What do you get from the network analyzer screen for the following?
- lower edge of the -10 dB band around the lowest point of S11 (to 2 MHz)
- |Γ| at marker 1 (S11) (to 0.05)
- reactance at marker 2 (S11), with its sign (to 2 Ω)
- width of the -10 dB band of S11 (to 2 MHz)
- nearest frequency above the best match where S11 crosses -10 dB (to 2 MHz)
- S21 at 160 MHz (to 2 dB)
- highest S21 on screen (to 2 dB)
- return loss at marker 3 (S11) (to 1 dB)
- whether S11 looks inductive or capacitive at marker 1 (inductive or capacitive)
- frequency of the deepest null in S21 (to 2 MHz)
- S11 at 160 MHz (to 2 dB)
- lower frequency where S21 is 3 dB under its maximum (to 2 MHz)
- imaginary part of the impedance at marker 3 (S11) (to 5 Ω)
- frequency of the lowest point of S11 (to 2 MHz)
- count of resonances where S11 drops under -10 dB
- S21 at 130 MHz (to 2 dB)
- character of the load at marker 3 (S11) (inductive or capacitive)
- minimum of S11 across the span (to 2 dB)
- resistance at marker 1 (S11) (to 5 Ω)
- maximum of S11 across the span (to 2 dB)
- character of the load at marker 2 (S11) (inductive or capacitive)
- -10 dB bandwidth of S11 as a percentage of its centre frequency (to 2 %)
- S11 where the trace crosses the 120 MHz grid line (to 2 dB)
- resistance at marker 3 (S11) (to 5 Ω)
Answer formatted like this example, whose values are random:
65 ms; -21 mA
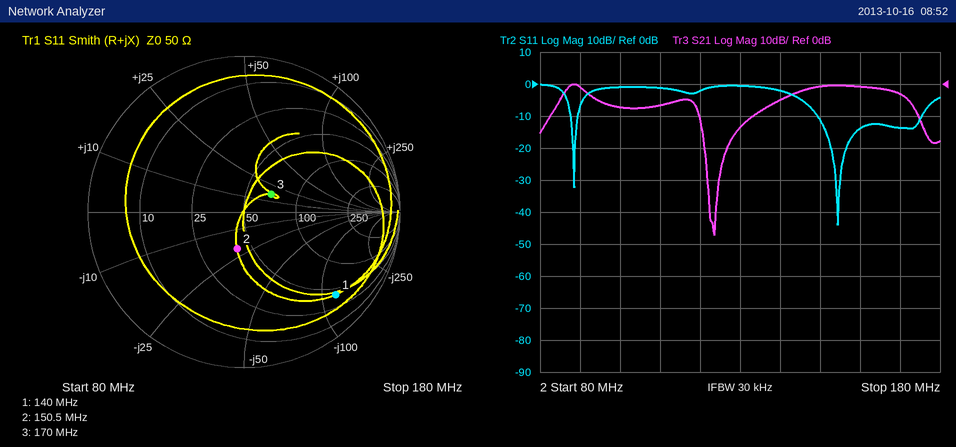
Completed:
150 MHz; 0.80; -20 Ω; 26 MHz; 176 MHz; 0 dB; 0 dB; 14 dB; capacitive; 124 MHz; -14 dB; 86 MHz; +15 Ω; 154 MHz; 2; -14 dB; inductive; -44 dB; 40 Ω; 0 dB; capacitive; 16 %; -2 dB; 70 Ω
